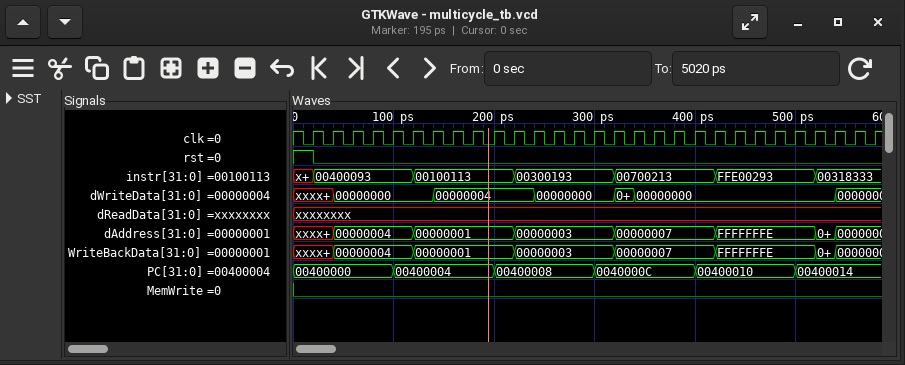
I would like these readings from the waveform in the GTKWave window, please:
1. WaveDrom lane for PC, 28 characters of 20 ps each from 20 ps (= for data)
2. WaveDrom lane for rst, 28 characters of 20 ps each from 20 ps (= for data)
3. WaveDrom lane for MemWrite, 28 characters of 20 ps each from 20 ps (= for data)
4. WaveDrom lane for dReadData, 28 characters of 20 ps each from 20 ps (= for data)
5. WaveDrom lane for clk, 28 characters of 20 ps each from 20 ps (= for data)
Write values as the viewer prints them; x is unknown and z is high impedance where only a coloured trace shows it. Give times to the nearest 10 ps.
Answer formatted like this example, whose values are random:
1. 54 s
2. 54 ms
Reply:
1. {name: 'PC', wave: '=...=....=....=....=....=...', data: '00400000 00400004 00400008 0040000C 00400010 00400014'}
2. {name: 'rst', wave: '0...........................'}
3. {name: 'MemWrite', wave: '0...........................'}
4. {name: 'dReadData', wave: 'x...........................'}
5. {name: 'clk', wave: 'p...........................'}
